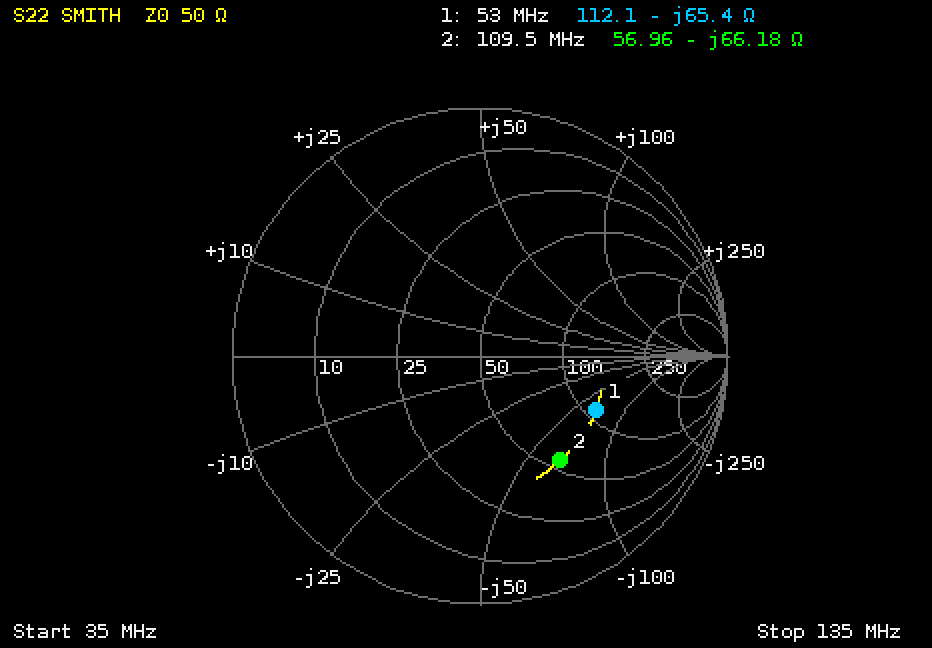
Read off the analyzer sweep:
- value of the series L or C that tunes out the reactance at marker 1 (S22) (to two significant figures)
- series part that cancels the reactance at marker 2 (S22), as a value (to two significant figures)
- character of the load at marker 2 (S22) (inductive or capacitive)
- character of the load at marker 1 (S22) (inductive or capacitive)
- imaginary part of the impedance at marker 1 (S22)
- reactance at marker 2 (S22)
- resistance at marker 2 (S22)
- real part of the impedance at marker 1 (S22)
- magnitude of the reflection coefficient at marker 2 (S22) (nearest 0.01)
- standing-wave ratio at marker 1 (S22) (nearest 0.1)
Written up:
200 nH
96 nH
capacitive
capacitive
-65.4 Ω
-66.18 Ω
56.96 Ω
112.1 Ω
0.53
3.1
